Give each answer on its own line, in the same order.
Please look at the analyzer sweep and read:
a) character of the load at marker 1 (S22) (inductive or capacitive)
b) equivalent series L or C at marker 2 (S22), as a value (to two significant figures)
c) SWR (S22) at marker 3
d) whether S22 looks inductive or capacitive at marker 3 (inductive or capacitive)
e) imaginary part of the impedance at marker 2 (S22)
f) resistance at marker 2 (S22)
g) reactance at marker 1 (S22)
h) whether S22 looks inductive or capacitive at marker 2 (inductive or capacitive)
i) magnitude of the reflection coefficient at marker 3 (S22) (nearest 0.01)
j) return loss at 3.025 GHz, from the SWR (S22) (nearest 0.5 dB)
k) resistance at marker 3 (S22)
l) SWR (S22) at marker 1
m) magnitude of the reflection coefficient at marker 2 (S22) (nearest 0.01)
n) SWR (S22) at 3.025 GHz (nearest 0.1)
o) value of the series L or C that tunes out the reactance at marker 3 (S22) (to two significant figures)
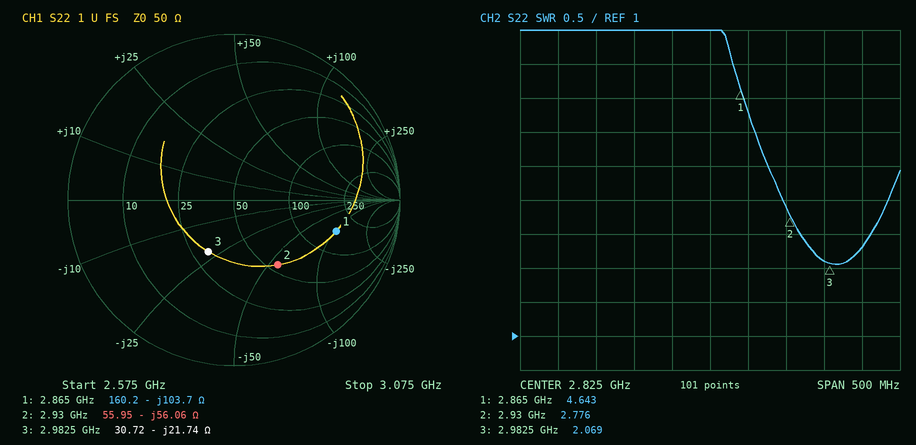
capacitive
970 fF
2.069
capacitive
-56.06 Ω
55.95 Ω
-103.7 Ω
capacitive
0.35
8.0 dB
30.72 Ω
4.643
0.47
2.3
1.2 nH
